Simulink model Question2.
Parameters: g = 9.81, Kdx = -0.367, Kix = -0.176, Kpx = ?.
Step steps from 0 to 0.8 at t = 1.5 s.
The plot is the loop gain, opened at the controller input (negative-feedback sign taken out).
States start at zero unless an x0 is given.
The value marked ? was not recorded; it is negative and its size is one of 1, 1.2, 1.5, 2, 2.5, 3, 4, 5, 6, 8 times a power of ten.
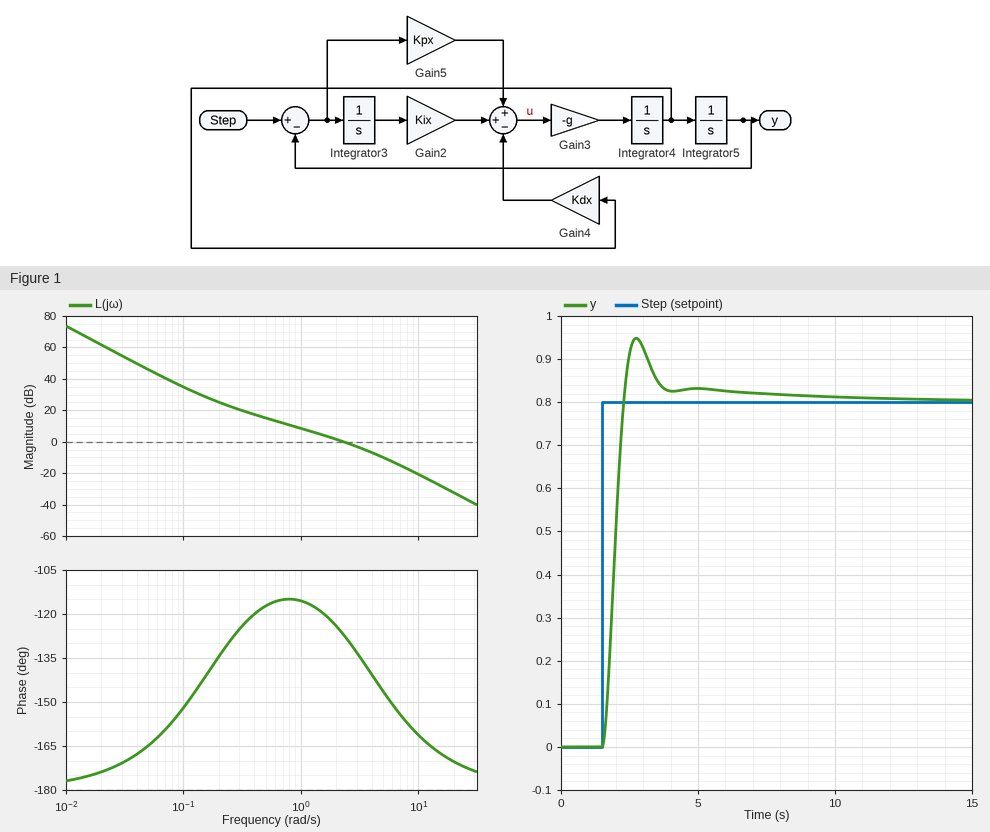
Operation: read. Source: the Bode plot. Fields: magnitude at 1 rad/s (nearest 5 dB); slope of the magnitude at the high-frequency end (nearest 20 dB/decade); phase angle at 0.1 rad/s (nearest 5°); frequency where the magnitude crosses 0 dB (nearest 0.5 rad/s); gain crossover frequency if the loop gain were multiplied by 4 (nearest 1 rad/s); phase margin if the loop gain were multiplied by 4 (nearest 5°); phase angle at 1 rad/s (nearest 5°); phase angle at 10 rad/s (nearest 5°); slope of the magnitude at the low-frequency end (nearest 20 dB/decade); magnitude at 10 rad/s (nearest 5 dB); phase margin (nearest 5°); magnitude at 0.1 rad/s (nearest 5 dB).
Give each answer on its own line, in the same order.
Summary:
10 dB
-40 dB/decade
-150°
2.5 rad/s
6 rad/s
30°
-115°
-160°
-40 dB/decade
-20 dB
55°
35 dB
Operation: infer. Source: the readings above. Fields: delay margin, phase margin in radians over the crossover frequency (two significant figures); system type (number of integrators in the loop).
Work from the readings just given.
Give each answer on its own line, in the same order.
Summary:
0.38 s
2
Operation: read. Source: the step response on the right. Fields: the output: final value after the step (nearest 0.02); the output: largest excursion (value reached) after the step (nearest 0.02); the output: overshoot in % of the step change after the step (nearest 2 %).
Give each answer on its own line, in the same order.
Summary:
0.80
0.94
18 %
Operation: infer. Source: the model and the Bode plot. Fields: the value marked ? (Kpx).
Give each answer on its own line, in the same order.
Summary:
-1
